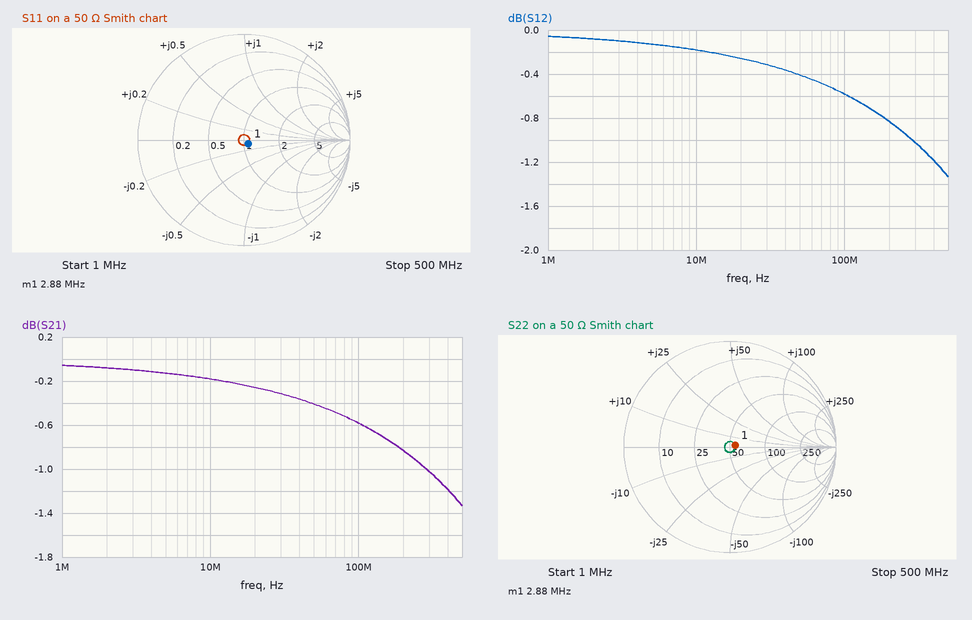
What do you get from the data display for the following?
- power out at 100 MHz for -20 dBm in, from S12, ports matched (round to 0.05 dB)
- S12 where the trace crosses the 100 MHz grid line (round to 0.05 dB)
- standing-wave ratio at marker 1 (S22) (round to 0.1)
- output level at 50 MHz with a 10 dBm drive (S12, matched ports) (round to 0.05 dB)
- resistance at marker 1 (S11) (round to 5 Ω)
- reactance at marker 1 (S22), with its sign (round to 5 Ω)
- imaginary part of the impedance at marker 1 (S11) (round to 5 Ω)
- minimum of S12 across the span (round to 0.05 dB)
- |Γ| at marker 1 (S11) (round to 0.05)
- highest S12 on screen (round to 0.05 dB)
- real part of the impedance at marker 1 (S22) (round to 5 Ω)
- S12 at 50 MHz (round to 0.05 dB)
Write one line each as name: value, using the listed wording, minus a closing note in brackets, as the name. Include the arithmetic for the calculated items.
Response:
power out at 100 MHz for -20 dBm in, from S12, ports matched: -20 dBm + (-0.60 dB) = -20.60 dBm
S12 where the trace crosses the 100 MHz grid line: -0.60 dB
standing-wave ratio at marker 1 (S22): 1.1
output level at 50 MHz with a 10 dBm drive (S12, matched ports): 10 dBm + (-0.40 dB) = 9.60 dBm
resistance at marker 1 (S11): 55 Ω
reactance at marker 1 (S22), with its sign: 0 Ω
imaginary part of the impedance at marker 1 (S11): -5 Ω
minimum of S12 across the span: -1.35 dB
|Γ| at marker 1 (S11): 0.05
highest S12 on screen: -0.05 dB
real part of the impedance at marker 1 (S22): 55 Ω
S12 at 50 MHz: -0.40 dB
